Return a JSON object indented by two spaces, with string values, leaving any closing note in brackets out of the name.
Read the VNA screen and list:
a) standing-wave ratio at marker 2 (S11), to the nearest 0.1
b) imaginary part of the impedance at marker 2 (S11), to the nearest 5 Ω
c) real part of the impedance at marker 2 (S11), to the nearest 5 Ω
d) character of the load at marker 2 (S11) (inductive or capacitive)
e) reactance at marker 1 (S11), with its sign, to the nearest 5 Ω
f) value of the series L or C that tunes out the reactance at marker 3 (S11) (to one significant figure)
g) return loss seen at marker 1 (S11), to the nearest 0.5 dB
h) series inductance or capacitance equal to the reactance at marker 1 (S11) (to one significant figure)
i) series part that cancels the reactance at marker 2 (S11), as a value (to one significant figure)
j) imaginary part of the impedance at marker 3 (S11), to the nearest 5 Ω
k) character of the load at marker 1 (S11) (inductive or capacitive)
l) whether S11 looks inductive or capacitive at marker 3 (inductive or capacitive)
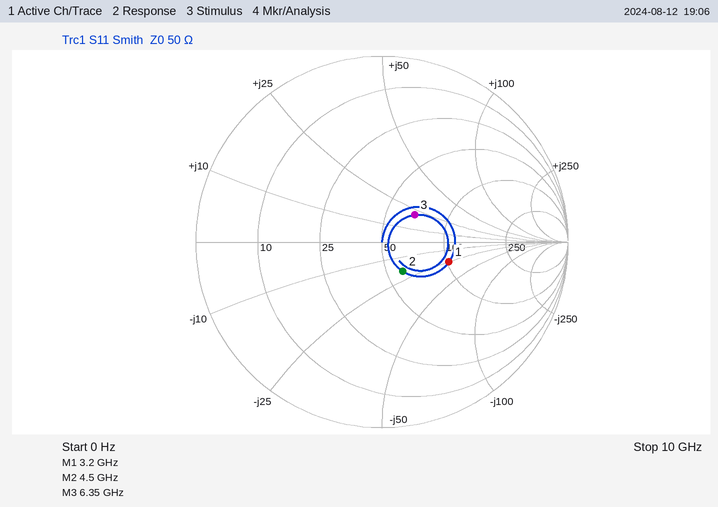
{
  "standing-wave ratio at marker 2 (S11), to the nearest 0.1": "1.5",
  "imaginary part of the impedance at marker 2 (S11), to the nearest 5 Ω": "-20 Ω",
  "real part of the impedance at marker 2 (S11), to the nearest 5 Ω": "60 Ω",
  "character of the load at marker 2 (S11)": "capacitive",
  "reactance at marker 1 (S11), with its sign, to the nearest 5 Ω": "-25 Ω",
  "value of the series L or C that tunes out the reactance at marker 3 (S11)": "1 pF",
  "return loss seen at marker 1 (S11), to the nearest 0.5 dB": "8.5 dB",
  "series inductance or capacitance equal to the reactance at marker 1 (S11)": "2 pF",
  "series part that cancels the reactance at marker 2 (S11), as a value": "700 pH",
  "imaginary part of the impedance at marker 3 (S11), to the nearest 5 Ω": "+20 Ω",
  "character of the load at marker 1 (S11)": "capacitive",
  "whether S11 looks inductive or capacitive at marker 3": "inductive"
}
